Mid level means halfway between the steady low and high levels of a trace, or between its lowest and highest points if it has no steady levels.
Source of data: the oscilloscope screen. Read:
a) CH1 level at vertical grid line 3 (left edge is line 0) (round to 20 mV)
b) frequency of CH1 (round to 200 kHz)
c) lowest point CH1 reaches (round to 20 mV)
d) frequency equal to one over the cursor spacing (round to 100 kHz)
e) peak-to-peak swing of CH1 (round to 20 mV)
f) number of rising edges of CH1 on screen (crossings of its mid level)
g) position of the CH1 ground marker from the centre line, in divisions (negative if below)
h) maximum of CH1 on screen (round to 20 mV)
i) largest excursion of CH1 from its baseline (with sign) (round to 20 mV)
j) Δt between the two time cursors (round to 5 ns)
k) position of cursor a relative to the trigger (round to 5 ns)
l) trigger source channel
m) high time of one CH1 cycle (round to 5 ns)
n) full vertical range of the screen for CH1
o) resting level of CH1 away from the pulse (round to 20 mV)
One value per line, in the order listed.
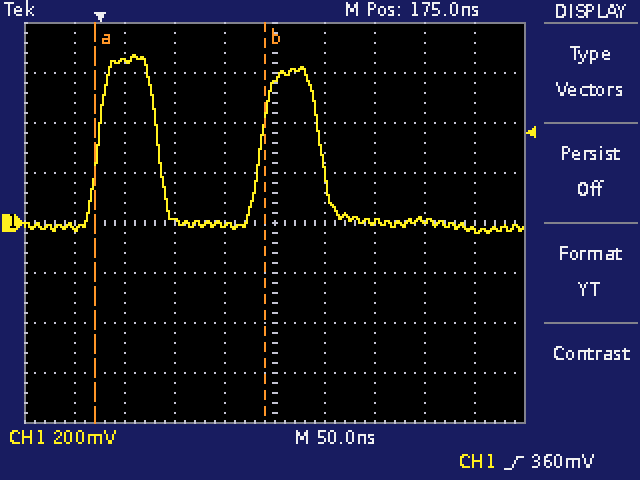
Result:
20 mV
6.2 MHz
-40 mV
5.9 MHz
720 mV
2
0.0 div
680 mV
+680 mV
170 ns
-5 ns
CH1
60 ns
1.6 V
0 mV
